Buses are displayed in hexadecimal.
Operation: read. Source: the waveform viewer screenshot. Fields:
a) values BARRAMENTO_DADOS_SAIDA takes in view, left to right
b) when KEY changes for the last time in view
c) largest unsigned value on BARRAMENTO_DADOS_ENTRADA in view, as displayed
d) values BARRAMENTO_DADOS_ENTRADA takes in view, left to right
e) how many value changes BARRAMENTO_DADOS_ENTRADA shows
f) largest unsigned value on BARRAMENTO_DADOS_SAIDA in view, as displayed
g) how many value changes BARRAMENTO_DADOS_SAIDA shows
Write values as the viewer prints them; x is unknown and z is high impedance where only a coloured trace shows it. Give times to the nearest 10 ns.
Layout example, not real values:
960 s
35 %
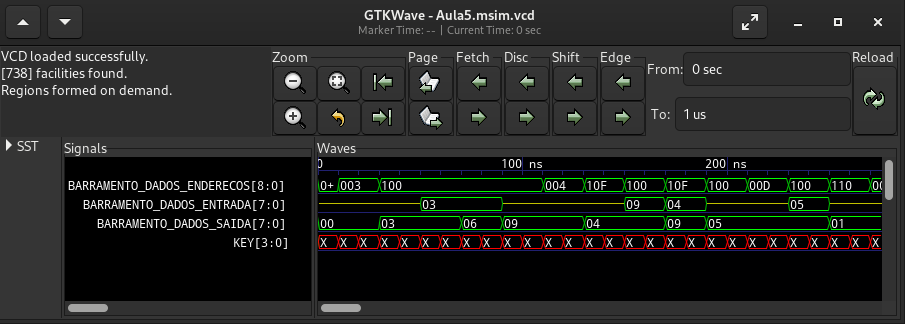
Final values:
00, 03, 06, 09, 04, 09, 05, 01
270 ns
09
z, 03, z, 09, 04, z, 05, z
7
09
7
